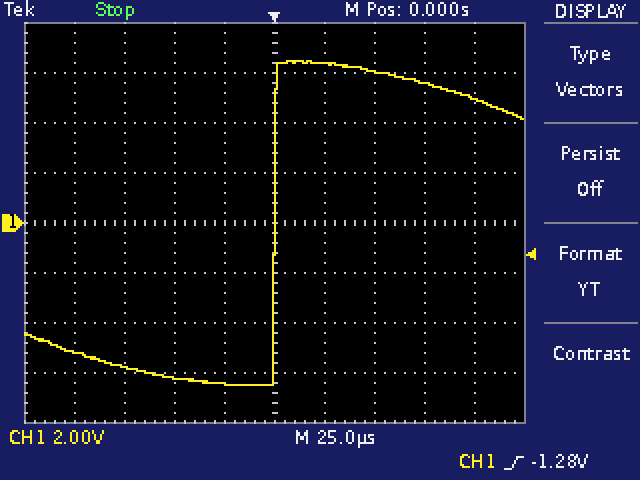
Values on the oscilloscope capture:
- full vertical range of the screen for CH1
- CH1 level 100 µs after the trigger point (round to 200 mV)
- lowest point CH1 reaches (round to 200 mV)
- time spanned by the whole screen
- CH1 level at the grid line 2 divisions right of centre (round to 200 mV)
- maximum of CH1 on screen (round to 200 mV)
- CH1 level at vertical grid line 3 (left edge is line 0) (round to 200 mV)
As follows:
16 V
5.0 V
-6.4 V
250 µs
6.0 V
6.4 V
-6.2 V
